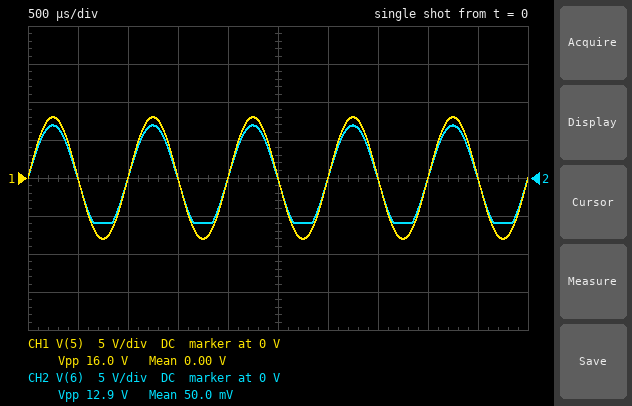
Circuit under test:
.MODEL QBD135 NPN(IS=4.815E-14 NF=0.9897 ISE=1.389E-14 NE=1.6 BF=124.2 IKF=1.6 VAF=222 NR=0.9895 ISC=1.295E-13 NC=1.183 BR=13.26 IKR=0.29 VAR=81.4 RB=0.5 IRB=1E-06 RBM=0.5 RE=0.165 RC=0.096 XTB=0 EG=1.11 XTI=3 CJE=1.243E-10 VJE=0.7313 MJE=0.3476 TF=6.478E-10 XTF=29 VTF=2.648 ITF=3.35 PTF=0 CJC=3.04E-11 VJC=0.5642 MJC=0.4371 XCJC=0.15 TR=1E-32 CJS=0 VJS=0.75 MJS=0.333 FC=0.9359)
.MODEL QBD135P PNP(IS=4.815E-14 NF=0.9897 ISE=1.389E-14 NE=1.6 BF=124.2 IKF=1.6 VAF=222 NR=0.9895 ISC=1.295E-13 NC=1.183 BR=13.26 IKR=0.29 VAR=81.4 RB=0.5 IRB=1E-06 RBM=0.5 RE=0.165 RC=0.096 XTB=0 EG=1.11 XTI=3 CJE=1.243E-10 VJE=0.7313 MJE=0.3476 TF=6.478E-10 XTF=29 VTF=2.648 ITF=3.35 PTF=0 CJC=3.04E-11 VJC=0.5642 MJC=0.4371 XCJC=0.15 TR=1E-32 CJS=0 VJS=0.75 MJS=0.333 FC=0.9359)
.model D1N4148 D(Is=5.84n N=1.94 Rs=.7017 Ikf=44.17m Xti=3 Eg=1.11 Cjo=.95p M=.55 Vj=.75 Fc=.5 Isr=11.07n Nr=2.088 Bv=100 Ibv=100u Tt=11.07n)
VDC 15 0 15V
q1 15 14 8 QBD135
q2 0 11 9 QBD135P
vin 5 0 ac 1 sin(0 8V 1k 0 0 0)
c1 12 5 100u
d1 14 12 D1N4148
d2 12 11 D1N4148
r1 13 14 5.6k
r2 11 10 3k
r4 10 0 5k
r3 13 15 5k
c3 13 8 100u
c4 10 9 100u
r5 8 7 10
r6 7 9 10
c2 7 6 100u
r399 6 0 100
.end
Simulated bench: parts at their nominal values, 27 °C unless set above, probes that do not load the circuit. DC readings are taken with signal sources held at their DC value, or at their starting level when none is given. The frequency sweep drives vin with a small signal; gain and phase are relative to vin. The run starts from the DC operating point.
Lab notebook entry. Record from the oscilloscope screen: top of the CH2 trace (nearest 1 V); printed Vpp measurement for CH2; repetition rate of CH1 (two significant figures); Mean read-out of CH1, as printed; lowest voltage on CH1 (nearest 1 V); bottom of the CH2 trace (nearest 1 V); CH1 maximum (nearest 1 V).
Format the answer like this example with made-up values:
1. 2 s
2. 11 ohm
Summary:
1. 7 V
2. 12.9 V
3. 1.0 kHz
4. 0.00 V
5. -8 V
6. -6 V
7. 8 V
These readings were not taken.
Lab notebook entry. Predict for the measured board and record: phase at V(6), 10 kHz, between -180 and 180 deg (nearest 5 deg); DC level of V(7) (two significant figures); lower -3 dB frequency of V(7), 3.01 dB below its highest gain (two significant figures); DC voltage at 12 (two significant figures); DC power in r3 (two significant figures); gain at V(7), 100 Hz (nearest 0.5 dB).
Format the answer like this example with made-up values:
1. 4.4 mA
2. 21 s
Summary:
1. 0 deg
2. 6.5 V
3. 300 mHz
4. 6.5 V
5. 2.8 mW
6. -3.5 dB
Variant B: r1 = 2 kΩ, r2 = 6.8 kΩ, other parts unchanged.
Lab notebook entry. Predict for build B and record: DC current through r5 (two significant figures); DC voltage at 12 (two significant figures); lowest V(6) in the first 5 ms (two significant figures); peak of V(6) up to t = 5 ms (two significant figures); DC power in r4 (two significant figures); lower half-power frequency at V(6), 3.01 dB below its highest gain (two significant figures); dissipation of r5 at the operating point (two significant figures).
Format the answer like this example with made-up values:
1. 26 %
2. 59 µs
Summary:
1. 300 µA
2. 9.3 V
3. -7.1 V
4. 5.2 V
5. 2.7 mW
6. 29 Hz
7. 930 nW
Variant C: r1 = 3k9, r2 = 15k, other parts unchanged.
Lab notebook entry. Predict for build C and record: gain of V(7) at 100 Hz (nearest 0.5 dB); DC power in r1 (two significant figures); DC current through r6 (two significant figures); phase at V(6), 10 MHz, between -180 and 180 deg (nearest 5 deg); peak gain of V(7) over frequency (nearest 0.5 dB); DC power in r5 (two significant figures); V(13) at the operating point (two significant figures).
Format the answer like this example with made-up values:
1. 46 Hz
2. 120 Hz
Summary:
1. -6.5 dB
2. 900 µW
3. 130 µA
4. 15 deg
5. 1.0 dB
6. 160 nW
7. 13 V
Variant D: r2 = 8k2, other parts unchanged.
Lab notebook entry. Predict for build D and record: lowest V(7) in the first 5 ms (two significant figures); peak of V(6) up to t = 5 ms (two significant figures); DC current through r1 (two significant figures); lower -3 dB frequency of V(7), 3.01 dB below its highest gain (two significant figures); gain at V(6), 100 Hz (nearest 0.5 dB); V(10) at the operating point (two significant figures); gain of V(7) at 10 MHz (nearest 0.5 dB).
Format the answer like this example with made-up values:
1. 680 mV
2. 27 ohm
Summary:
1. 1.8 V
2. 6.0 V
3. 580 µA
4. 230 mHz
5. -5.0 dB
6. 2.9 V
7. -4.5 dB
